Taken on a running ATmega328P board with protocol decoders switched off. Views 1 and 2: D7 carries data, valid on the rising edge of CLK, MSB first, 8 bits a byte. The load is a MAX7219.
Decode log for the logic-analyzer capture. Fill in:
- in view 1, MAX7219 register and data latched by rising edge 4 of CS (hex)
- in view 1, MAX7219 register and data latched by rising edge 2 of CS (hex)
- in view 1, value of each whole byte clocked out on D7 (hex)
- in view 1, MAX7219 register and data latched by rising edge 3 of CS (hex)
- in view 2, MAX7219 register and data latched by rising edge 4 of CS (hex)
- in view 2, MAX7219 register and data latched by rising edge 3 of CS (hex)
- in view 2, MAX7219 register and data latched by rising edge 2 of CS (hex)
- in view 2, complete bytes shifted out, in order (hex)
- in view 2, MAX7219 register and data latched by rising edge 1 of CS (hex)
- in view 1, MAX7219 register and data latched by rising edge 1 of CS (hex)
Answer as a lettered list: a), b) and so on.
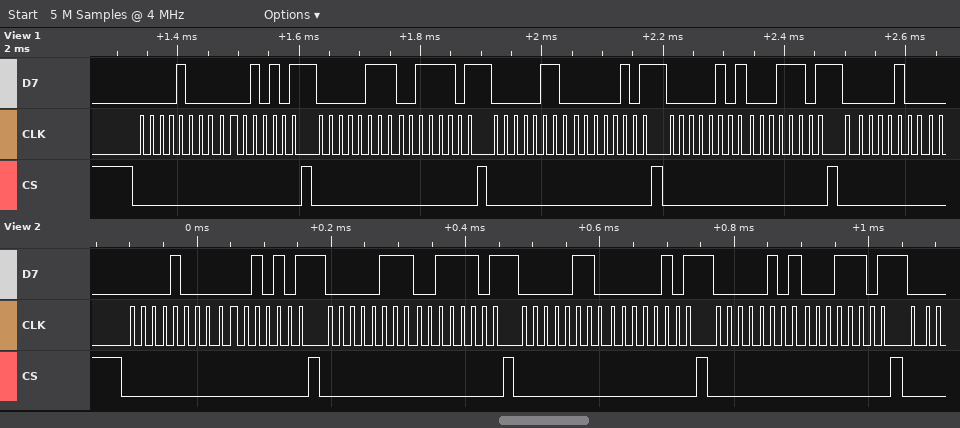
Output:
a) register 0x5, data 0x1D
b) register 0x7, data 0x3D
c) 08 15 07 3D 06 05 05 1D 04
d) register 0x6, data 0x05
e) register 0x5, data 0x1D
f) register 0x6, data 0x05
g) register 0x7, data 0x3D
h) 08 15 07 3D 06 05 05 1D
i) register 0x8, data 0x15
j) register 0x8, data 0x15
